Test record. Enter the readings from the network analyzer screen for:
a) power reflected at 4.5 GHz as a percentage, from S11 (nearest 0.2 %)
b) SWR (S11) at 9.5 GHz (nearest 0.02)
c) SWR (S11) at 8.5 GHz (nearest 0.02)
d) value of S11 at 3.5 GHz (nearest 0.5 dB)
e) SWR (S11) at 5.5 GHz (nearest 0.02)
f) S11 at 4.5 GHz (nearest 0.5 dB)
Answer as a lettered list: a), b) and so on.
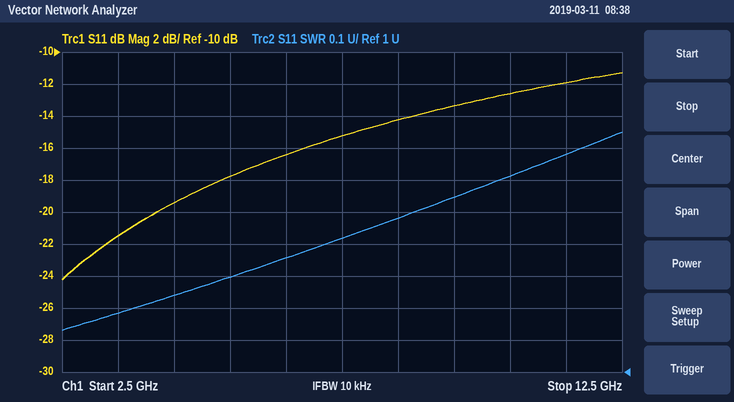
a) 1.2 %
b) 1.54
c) 1.48
d) -21.5 dB
e) 1.30
f) -19.5 dB
